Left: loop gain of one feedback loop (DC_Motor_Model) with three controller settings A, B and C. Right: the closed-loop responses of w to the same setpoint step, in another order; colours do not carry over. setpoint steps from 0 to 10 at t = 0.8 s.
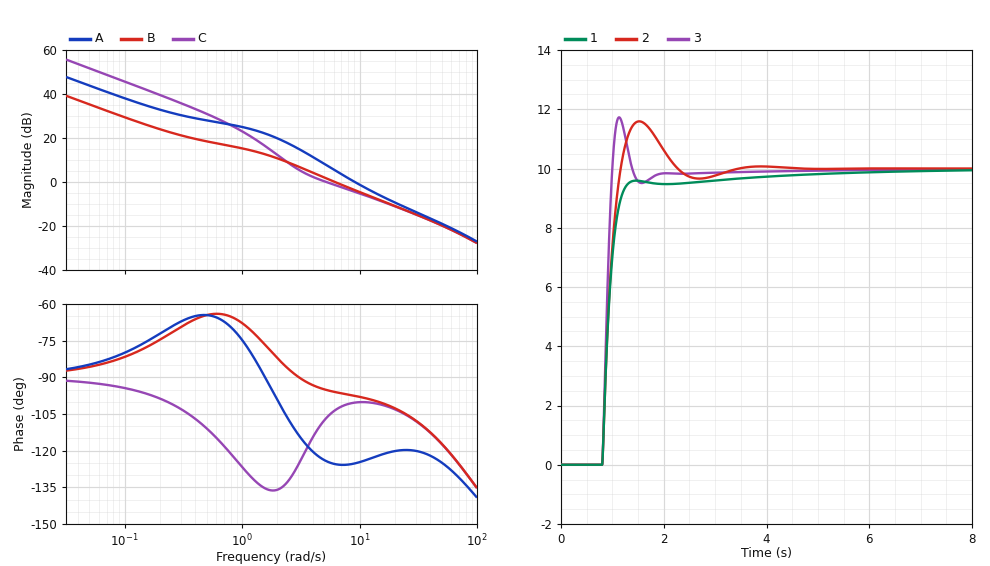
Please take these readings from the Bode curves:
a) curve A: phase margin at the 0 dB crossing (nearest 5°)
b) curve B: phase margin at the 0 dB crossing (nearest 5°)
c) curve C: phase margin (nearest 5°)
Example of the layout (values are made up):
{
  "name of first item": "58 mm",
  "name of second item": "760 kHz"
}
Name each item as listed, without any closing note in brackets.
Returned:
{
  "curve A: phase margin at the 0 dB crossing": "55°",
  "curve B: phase margin at the 0 dB crossing": "85°",
  "curve C: phase margin": "75°"
}
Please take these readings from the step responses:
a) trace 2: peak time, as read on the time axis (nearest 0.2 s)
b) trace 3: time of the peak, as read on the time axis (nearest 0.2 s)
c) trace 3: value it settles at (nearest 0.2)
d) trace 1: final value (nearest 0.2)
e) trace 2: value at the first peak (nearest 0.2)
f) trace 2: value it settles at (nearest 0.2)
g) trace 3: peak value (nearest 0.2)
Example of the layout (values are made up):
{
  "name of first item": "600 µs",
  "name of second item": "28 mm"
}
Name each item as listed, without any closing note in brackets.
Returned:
{
  "trace 2: peak time, as read on the time axis": "1.6 s",
  "trace 3: time of the peak, as read on the time axis": "1.2 s",
  "trace 3: value it settles at": "10.0",
  "trace 1: final value": "10.0",
  "trace 2: value at the first peak": "11.6",
  "trace 2: value it settles at": "10.0",
  "trace 3: peak value": "11.8"
}
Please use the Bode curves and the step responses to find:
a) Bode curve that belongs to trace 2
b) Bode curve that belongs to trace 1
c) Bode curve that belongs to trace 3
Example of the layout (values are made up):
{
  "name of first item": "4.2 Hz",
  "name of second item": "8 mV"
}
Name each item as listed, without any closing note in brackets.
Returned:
{
  "Bode curve that belongs to trace 2": "C",
  "Bode curve that belongs to trace 1": "B",
  "Bode curve that belongs to trace 3": "A"
}
